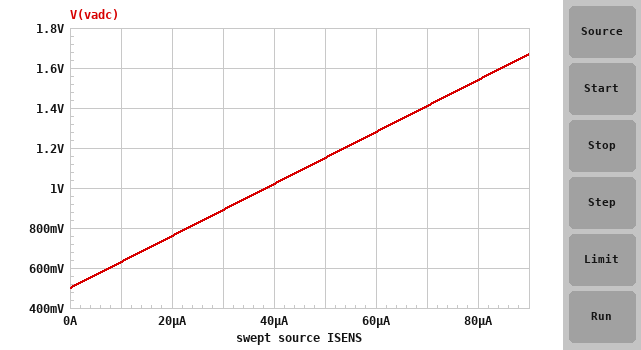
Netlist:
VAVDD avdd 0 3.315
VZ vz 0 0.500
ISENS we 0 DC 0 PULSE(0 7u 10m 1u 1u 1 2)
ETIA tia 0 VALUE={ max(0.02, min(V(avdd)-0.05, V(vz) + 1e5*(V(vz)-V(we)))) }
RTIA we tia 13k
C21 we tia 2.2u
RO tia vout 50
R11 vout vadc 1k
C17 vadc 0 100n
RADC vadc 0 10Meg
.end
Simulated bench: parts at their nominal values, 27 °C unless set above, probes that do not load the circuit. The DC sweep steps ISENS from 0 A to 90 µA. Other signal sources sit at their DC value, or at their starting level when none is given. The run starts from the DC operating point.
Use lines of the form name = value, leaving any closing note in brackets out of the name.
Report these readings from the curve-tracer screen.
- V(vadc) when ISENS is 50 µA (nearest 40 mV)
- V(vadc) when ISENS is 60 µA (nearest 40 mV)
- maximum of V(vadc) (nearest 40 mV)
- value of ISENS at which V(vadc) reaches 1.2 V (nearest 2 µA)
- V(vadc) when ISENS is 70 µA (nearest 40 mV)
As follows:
V(vadc) when ISENS is 50 µA = 1.16 V
V(vadc) when ISENS is 60 µA = 1.28 V
maximum of V(vadc) = 1.68 V
value of ISENS at which V(vadc) reaches 1.2 V = 54 µA
V(vadc) when ISENS is 70 µA = 1.40 V
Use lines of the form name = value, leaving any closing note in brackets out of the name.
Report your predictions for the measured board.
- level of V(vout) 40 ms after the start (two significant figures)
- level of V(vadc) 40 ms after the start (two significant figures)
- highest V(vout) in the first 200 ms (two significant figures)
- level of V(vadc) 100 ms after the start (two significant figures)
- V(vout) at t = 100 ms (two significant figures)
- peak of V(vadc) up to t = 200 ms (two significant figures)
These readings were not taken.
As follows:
level of V(vout) 40 ms after the start = 560 mV
level of V(vadc) 40 ms after the start = 560 mV
highest V(vout) in the first 200 ms = 590 mV
level of V(vadc) 100 ms after the start = 590 mV
V(vout) at t = 100 ms = 590 mV
peak of V(vadc) up to t = 200 ms = 590 mV
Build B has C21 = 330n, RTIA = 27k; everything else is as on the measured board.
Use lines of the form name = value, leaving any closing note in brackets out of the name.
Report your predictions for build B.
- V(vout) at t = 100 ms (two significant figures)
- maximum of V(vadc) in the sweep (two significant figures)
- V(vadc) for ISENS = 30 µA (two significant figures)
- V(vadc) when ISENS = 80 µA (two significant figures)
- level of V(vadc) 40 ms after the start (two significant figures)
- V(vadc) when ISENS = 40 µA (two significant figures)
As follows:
V(vout) at t = 100 ms = 690 mV
maximum of V(vadc) in the sweep = 2.9 V
V(vadc) for ISENS = 30 µA = 1.3 V
V(vadc) when ISENS = 80 µA = 2.7 V
level of V(vadc) 40 ms after the start = 680 mV
V(vadc) when ISENS = 40 µA = 1.6 V
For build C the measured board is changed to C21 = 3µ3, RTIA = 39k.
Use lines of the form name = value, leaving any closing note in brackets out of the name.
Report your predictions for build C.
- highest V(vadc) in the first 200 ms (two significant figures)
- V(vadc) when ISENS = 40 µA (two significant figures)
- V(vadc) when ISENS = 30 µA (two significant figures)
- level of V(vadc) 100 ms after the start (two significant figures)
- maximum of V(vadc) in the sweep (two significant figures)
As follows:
highest V(vadc) in the first 200 ms = 710 mV
V(vadc) when ISENS = 40 µA = 2.1 V
V(vadc) when ISENS = 30 µA = 1.7 V
level of V(vadc) 100 ms after the start = 640 mV
maximum of V(vadc) in the sweep = 3.3 V
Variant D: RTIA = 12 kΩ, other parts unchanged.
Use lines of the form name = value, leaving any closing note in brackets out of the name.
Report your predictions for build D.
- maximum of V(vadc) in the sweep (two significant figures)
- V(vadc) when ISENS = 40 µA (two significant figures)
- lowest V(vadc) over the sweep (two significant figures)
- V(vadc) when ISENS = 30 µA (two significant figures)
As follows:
maximum of V(vadc) in the sweep = 1.6 V
V(vadc) when ISENS = 40 µA = 980 mV
lowest V(vadc) over the sweep = 500 mV
V(vadc) when ISENS = 30 µA = 860 mV
